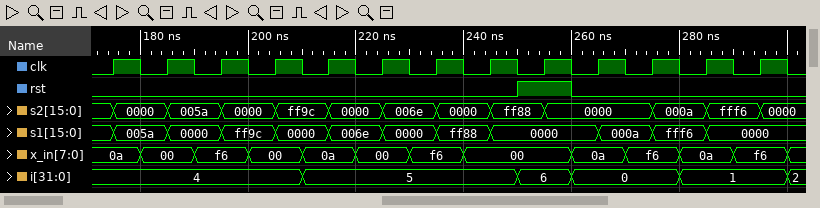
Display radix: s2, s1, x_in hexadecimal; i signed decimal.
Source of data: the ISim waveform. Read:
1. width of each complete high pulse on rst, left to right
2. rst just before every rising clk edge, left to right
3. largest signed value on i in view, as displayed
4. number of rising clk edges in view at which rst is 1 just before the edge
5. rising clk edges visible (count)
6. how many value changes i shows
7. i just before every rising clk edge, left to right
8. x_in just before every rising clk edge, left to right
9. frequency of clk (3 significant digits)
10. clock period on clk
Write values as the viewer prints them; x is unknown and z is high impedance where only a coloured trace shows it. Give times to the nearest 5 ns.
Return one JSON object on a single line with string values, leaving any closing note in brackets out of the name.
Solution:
{"width of each complete high pulse on rst, left to right": "10 ns", "rst just before every rising clk edge, left to right": "0 0 0 0 0 0 0 0 1 0 0 0 0", "largest signed value on i in view, as displayed": "6", "number of rising clk edges in view at which rst is 1 just before the edge": "1", "rising clk edges visible": "13", "how many value changes i shows": "5", "i just before every rising clk edge, left to right": "4, 4, 4, 4, 5, 5, 5, 5, 6, 0, 0, 1, 1", "x_in just before every rising clk edge, left to right": "0a, 00, f6, 00, 0a, 00, f6, 00, 00, 0a, f6, 0a, f6", "frequency of clk": "100 MHz", "clock period on clk": "10 ns"}
